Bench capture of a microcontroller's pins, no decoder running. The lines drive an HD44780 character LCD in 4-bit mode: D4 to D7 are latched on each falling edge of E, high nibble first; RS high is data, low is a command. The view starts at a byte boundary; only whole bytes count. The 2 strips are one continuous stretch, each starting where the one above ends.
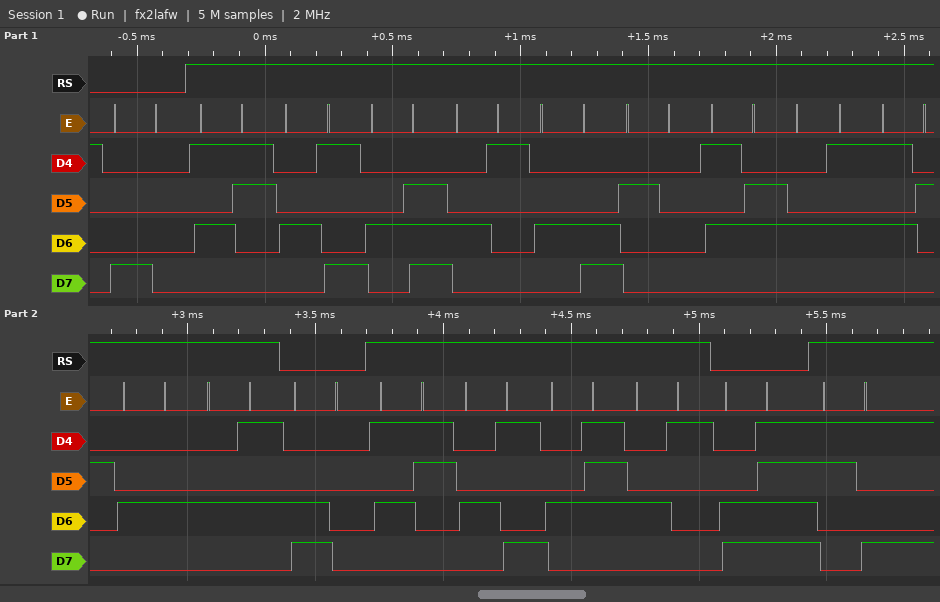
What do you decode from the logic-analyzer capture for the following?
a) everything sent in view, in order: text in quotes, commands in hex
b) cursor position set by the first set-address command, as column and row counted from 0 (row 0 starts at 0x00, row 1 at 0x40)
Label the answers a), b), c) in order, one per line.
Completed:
a) 0x80 "SINAL VERDE" 0xC0 "SIGA" 0xCF "9"
b) column 0, row 0
